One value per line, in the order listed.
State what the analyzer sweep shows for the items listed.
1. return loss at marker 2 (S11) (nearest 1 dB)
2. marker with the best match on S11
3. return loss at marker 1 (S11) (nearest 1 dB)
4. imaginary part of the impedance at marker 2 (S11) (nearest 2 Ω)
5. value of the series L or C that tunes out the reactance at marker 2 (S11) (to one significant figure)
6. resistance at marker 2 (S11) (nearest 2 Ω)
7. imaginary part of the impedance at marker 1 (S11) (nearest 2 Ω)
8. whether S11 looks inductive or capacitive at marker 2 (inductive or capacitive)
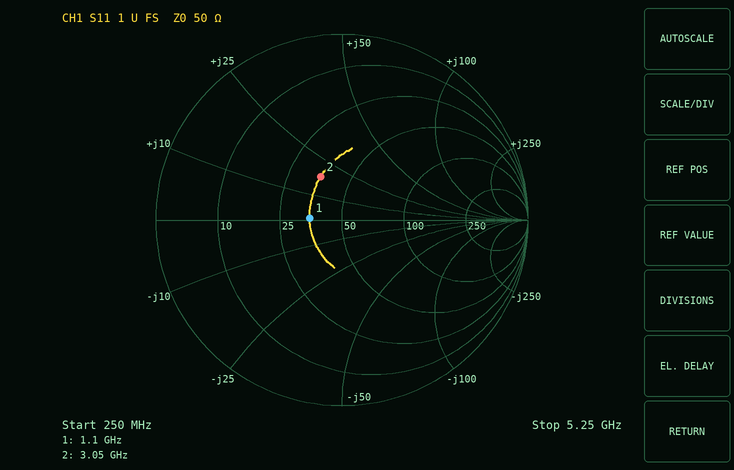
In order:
12 dB
marker 1
15 dB
+18 Ω
3 pF
36 Ω
0 Ω
inductive
